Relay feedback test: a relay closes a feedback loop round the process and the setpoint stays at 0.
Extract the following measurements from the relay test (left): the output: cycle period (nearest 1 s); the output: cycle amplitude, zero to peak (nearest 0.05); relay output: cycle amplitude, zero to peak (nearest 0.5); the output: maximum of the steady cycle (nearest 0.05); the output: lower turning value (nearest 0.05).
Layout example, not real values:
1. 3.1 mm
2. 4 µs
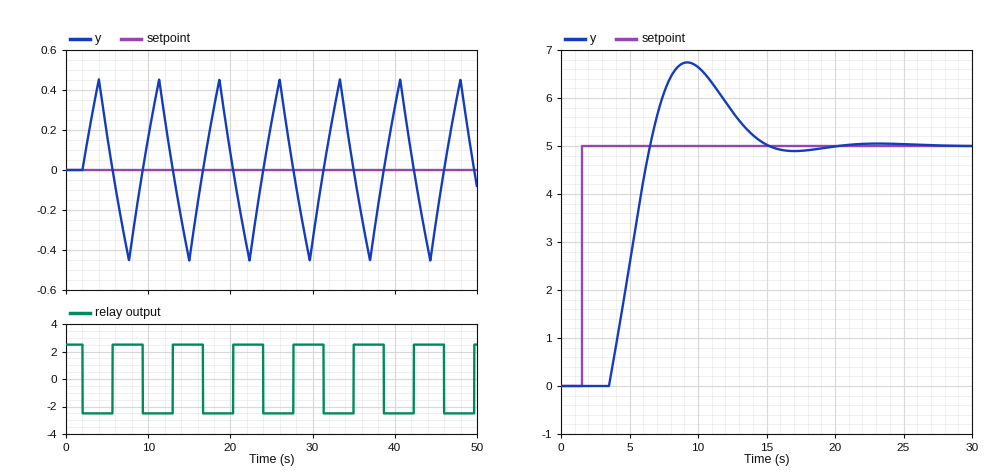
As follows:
1. 7 s
2. 0.45
3. 2.5
4. 0.45
5. -0.45
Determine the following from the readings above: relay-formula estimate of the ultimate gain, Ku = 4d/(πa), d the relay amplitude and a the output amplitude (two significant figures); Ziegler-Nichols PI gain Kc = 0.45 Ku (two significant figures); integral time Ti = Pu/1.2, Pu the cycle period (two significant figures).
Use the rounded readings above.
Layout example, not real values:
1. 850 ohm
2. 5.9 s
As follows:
1. 7.1
2. 3.2
3. 5.8 s
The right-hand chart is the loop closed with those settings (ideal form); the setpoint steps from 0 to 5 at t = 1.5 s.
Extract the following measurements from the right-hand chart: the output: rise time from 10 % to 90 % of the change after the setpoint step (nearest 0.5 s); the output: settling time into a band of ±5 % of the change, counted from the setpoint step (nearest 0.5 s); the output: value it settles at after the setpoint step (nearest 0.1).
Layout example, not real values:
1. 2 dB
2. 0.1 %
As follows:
1. 2.5 s
2. 12.5 s
3. 5.0
